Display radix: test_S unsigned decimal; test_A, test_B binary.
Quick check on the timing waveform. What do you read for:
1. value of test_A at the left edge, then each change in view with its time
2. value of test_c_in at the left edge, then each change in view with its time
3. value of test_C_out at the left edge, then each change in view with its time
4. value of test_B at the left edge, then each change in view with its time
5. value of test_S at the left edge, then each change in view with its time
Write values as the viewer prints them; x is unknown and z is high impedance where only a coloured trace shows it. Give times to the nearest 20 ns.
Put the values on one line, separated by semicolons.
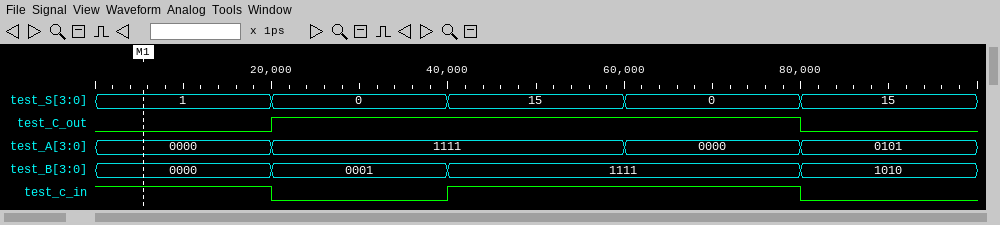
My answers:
0000, 1111 at 20 ns, 0000 at 60 ns, 0101 at 80 ns; 1, 0 at 20 ns, 1 at 40 ns, 0 at 80 ns; 0, 1 at 20 ns, 0 at 80 ns; 0000, 0001 at 20 ns, 1111 at 40 ns, 1010 at 80 ns; 1, 0 at 20 ns, 15 at 40 ns, 0 at 60 ns, 15 at 80 ns
